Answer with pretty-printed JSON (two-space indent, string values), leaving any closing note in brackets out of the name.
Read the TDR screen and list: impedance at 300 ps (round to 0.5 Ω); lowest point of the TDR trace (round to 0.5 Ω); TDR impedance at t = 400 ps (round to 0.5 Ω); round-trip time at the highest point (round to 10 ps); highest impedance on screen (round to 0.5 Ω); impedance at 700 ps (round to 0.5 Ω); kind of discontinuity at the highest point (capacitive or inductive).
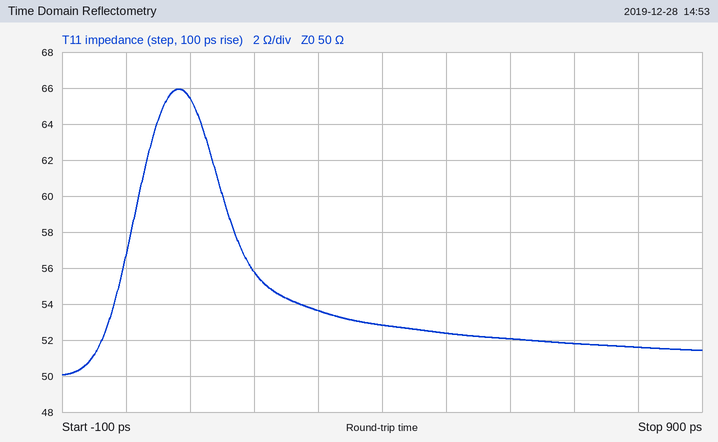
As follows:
{
  "impedance at 300 ps": "53.5 Ω",
  "lowest point of the TDR trace": "50.0 Ω",
  "TDR impedance at t = 400 ps": "53.0 Ω",
  "round-trip time at the highest point": "80 ps",
  "highest impedance on screen": "66.0 Ω",
  "impedance at 700 ps": "52.0 Ω",
  "kind of discontinuity at the highest point": "inductive"
}
